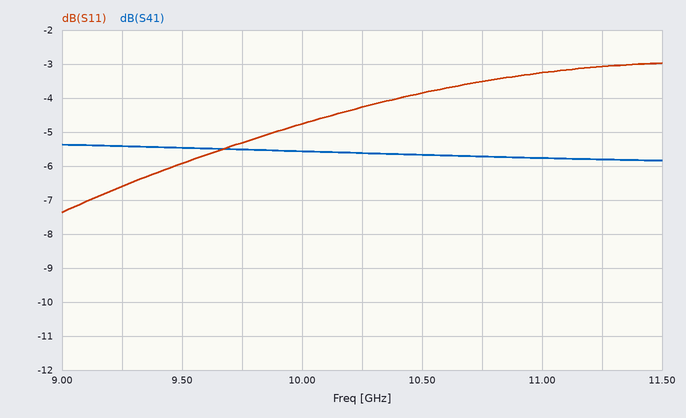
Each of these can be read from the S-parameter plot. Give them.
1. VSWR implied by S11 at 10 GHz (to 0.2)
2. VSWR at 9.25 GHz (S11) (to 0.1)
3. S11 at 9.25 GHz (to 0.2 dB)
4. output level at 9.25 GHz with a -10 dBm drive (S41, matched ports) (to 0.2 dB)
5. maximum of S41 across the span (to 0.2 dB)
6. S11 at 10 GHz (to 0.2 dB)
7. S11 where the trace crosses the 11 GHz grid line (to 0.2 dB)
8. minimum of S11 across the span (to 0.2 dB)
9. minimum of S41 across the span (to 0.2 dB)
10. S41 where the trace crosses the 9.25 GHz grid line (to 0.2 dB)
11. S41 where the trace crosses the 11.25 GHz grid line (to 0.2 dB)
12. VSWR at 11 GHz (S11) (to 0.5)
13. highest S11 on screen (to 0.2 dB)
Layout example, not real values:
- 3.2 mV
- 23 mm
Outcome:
- 3.8
- 2.8
- -6.6 dB
- -15.4 dBm
- -5.4 dB
- -4.8 dB
- -3.2 dB
- -7.4 dB
- -5.8 dB
- -5.4 dB
- -5.8 dB
- 5.5
- -3.0 dB
